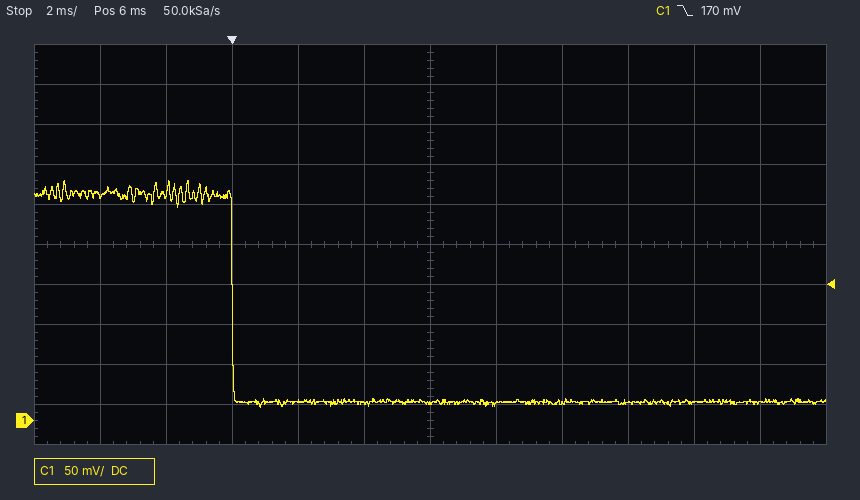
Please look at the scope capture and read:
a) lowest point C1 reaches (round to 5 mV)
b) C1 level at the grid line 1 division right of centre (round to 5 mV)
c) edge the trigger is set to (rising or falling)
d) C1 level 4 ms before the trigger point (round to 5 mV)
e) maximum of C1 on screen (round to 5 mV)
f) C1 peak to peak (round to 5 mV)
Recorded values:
15 mV
20 mV
falling
280 mV
300 mV
285 mV
